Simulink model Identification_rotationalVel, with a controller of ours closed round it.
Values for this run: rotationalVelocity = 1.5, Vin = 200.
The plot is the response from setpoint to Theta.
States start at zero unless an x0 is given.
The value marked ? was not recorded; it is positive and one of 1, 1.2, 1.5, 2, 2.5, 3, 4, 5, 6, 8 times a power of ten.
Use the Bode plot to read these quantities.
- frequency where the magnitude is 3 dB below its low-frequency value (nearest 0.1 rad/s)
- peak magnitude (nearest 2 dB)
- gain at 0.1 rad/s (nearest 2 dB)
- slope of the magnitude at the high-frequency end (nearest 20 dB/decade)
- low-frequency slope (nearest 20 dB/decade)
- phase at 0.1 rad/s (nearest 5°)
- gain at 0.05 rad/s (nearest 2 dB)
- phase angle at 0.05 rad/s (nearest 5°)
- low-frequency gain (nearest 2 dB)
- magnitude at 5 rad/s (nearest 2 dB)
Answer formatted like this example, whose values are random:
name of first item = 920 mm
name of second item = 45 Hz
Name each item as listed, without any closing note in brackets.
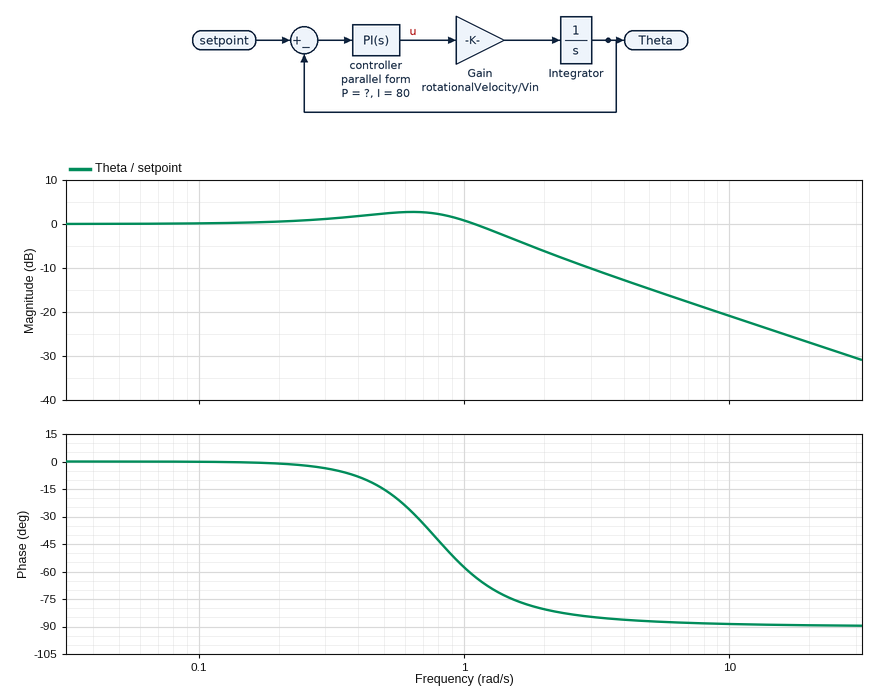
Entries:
frequency where the magnitude is 3 dB below its low-frequency value = 1.5 rad/s
peak magnitude = 2 dB
gain at 0.1 rad/s = 0 dB
slope of the magnitude at the high-frequency end = -20 dB/decade
low-frequency slope = 0 dB/decade
phase at 0.1 rad/s = 0°
gain at 0.05 rad/s = 0 dB
phase angle at 0.05 rad/s = 0°
low-frequency gain = 0 dB
magnitude at 5 rad/s = -14 dB
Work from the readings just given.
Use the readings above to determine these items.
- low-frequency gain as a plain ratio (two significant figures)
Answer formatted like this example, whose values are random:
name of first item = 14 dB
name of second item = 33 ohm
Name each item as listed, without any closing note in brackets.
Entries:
low-frequency gain as a plain ratio = 1.0
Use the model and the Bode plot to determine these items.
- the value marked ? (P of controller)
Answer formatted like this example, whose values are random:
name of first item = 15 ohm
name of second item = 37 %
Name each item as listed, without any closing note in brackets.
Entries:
the value marked ? = 120
